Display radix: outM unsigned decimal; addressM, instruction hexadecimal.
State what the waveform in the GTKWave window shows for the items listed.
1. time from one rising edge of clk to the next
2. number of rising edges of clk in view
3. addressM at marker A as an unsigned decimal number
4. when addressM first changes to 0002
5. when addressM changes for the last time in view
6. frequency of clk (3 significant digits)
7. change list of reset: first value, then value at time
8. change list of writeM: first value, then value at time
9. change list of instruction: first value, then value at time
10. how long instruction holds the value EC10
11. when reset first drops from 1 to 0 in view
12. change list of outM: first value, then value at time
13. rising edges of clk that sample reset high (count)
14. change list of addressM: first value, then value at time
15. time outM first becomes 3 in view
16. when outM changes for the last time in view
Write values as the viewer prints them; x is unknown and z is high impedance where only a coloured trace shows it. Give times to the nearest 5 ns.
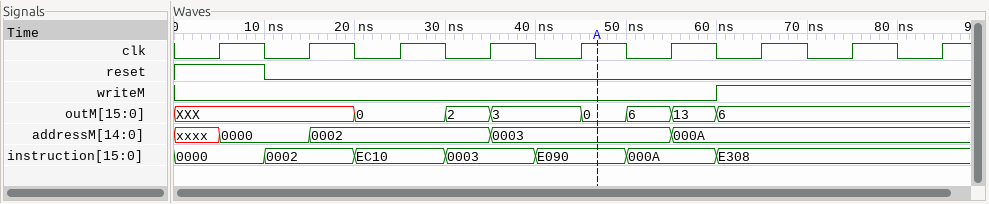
10 ns
9
3
15 ns
55 ns
100 MHz
1, 0 at 10 ns
0, 1 at 60 ns
0000, 0002 at 10 ns, EC10 at 20 ns, 0003 at 30 ns, E090 at 40 ns, 000A at 50 ns, E308 at 60 ns
10 ns
10 ns
XXX, 0 at 20 ns, 2 at 30 ns, 3 at 35 ns, 0 at 45 ns, 6 at 50 ns, 13 at 55 ns, 6 at 60 ns
1
xxxx, 0000 at 5 ns, 0002 at 15 ns, 0003 at 35 ns, 000A at 55 ns
35 ns
60 ns
